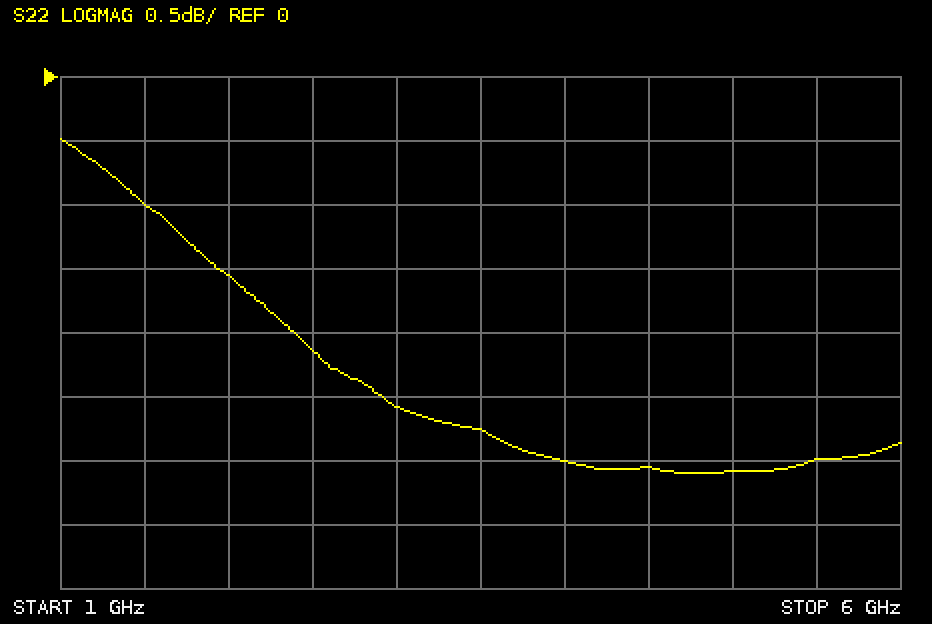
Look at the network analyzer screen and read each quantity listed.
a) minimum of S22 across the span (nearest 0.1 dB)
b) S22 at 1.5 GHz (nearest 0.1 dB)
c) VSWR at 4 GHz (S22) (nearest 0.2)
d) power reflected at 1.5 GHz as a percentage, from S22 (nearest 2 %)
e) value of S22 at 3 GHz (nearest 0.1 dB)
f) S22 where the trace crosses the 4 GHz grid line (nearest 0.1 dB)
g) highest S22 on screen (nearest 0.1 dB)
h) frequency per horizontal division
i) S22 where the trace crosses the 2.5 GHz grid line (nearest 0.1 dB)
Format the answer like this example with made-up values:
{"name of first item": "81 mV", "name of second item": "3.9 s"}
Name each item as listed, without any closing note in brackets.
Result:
{"minimum of S22 across the span": "-3.1 dB", "S22 at 1.5 GHz": "-1.0 dB", "VSWR at 4 GHz (S22)": "5.8", "power reflected at 1.5 GHz as a percentage, from S22": "80 %", "value of S22 at 3 GHz": "-2.6 dB", "S22 where the trace crosses the 4 GHz grid line": "-3.0 dB", "highest S22 on screen": "-0.5 dB", "frequency per horizontal division": "500 MHz", "S22 where the trace crosses the 2.5 GHz grid line": "-2.1 dB"}
